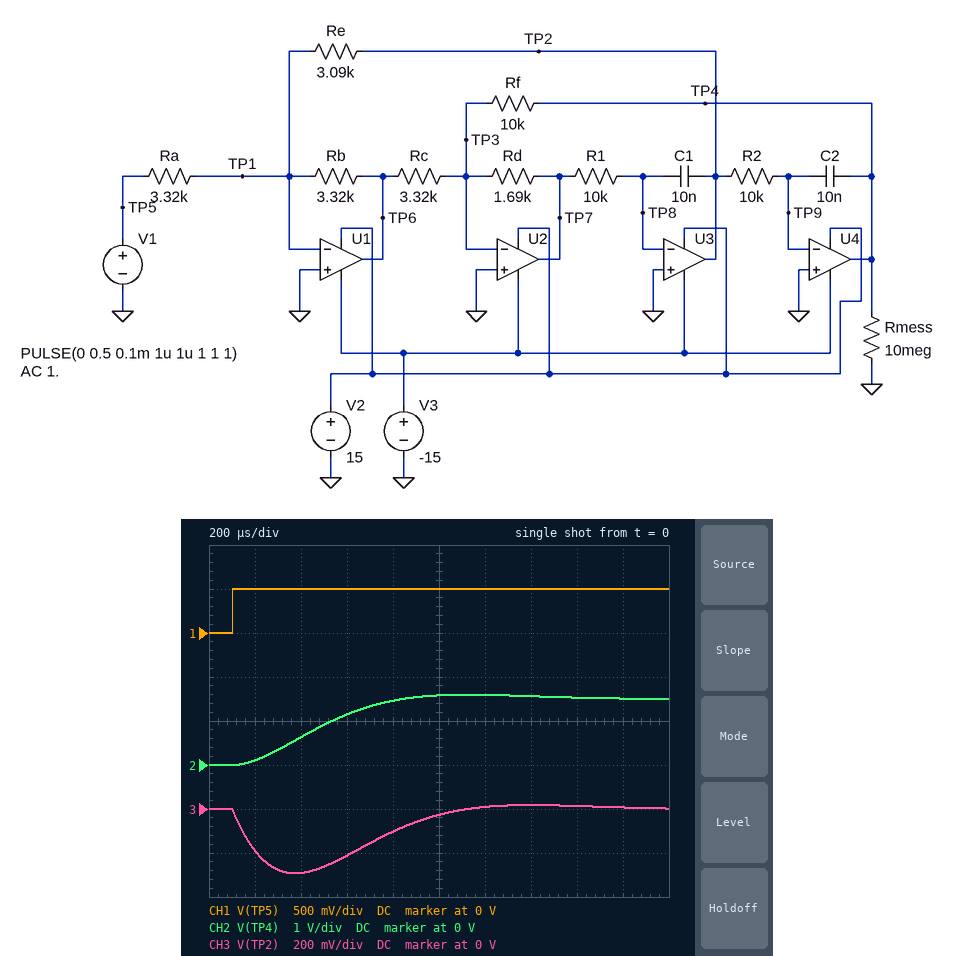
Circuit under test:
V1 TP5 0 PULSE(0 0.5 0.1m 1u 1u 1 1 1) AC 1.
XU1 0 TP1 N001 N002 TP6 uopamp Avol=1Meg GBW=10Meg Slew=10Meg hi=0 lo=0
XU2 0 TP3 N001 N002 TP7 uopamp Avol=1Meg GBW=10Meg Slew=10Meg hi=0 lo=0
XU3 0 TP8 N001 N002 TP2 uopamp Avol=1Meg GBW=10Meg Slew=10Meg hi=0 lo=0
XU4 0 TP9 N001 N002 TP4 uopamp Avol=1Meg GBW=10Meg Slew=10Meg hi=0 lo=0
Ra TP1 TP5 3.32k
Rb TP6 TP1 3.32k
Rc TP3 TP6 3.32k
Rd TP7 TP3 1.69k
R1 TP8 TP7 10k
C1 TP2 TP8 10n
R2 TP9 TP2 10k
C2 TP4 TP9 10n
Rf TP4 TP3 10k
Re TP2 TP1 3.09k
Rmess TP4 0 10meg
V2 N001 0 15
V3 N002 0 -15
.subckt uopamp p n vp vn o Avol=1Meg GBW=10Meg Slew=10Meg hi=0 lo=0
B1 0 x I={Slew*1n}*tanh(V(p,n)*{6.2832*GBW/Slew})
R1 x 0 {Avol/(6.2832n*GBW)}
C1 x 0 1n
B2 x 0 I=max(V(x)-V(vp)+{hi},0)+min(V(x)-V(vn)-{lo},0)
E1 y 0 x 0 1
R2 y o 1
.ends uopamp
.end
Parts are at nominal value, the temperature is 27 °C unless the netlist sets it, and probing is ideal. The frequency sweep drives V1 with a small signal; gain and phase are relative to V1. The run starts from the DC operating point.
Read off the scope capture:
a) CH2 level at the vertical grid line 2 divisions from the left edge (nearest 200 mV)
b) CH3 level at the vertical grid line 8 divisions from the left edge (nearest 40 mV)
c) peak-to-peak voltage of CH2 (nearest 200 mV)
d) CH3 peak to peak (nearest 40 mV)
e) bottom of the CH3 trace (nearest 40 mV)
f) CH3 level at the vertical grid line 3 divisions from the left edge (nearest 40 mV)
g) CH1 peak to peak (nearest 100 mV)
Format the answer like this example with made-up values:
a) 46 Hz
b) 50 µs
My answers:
a) 600 mV
b) 0 V
c) 1.6 V
d) 320 mV
e) -280 mV
f) -200 mV
g) 500 mV
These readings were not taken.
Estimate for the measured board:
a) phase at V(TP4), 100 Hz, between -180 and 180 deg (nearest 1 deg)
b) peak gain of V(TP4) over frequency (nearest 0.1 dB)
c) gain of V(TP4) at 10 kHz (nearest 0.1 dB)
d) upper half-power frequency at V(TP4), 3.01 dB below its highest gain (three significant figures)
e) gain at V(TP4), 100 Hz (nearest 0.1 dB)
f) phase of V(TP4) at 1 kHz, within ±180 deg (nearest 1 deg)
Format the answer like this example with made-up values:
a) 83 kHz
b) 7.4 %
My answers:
a) -12 deg
b) 9.6 dB
c) -37.8 dB
d) 689 Hz
e) 9.6 dB
f) -123 deg
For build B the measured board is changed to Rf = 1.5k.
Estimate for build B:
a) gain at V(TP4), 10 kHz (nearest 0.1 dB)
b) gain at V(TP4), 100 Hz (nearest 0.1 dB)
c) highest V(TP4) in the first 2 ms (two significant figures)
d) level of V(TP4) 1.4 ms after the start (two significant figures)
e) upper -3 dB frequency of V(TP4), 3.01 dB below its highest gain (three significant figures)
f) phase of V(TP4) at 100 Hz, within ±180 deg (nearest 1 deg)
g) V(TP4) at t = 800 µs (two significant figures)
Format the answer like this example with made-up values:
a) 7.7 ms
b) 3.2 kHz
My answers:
a) -37.6 dB
b) -6.9 dB
c) 320 mV
d) 220 mV
e) 1.97 kHz
f) -2 deg
g) 200 mV
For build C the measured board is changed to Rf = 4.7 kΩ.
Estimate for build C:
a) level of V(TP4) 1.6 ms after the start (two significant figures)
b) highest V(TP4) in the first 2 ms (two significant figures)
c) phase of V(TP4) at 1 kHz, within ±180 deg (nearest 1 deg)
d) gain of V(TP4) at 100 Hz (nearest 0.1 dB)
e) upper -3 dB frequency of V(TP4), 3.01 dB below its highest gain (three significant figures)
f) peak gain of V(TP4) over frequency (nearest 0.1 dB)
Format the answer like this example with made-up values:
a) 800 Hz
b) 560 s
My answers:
a) 700 mV
b) 850 mV
c) -96 deg
d) 3.1 dB
e) 1.13 kHz
f) 4.8 dB
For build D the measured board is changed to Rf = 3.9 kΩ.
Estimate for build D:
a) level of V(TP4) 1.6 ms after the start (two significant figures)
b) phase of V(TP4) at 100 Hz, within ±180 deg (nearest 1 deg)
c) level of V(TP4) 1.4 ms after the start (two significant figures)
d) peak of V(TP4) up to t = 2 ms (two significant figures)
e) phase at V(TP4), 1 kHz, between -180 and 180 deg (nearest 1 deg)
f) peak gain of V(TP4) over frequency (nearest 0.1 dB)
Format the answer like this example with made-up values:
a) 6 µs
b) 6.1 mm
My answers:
a) 590 mV
b) -5 deg
c) 580 mV
d) 730 mV
e) -84 deg
f) 3.8 dB
